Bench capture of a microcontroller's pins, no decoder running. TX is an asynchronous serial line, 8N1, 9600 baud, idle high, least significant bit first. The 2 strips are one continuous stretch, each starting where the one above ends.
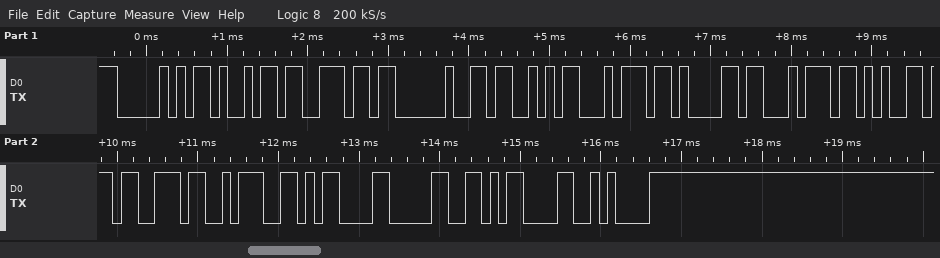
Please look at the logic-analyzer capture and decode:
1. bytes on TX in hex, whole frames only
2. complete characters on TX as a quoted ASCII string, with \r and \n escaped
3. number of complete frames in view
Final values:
0x50 0x69 0x6E 0x20 0x53 0x74 0x61 0x74 0x65 0x73 0x3A 0x0D 0x30 0x0D 0x0A
"Pin States:\r0\r\n"
15
